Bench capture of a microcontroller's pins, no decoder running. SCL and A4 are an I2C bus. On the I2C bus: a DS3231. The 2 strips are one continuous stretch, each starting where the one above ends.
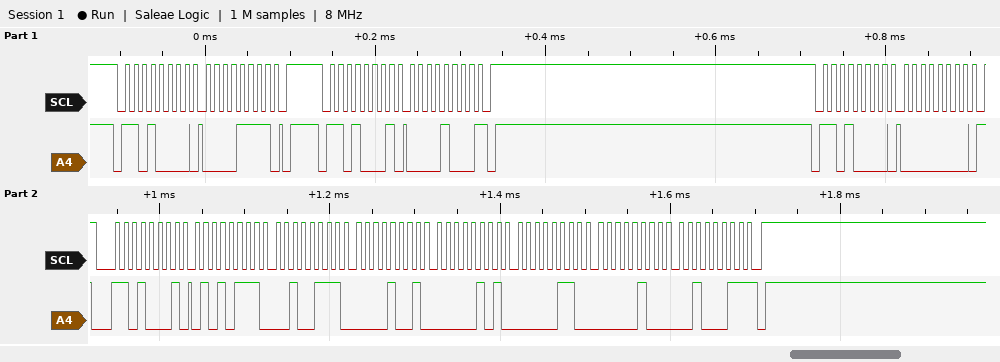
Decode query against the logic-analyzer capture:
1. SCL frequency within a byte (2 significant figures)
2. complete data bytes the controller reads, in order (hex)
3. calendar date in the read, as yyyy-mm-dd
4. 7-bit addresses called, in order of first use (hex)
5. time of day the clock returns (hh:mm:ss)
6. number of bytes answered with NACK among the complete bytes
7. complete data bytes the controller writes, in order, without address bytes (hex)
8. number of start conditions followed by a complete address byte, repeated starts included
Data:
100 kHz
08 57 27 09 05 06 04 23
2023-04-06
0x68
09:27:57
2
0F 00
4
